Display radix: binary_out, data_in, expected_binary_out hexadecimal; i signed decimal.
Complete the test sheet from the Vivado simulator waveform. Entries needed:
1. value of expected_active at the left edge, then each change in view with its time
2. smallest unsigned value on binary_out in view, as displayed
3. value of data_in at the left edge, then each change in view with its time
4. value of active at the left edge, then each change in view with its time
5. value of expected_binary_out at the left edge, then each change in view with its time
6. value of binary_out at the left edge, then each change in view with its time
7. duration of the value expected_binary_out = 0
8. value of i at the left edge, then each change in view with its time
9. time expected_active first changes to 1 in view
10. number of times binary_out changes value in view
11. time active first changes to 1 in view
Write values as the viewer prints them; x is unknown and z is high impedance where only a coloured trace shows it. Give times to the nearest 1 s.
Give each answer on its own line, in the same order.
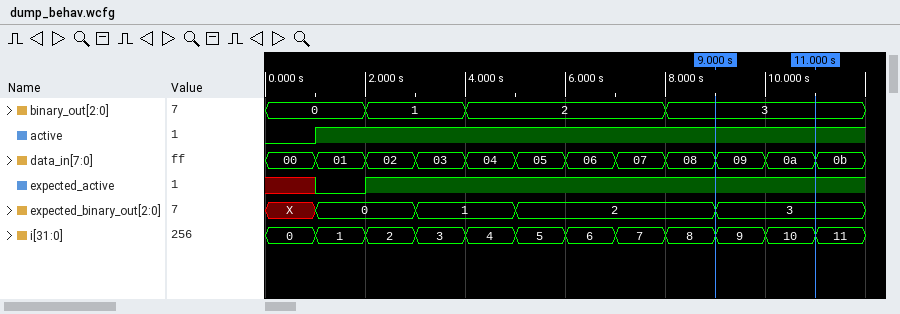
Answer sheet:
x, 0 at 1 s, 1 at 2 s
0
00, 01 at 1 s, 02 at 2 s, 03 at 3 s, 04 at 4 s, 05 at 5 s, 06 at 6 s, 07 at 7 s, 08 at 8 s, 09 at 9 s, 0a at 10 s, 0b at 11 s
0, 1 at 1 s
X, 0 at 1 s, 1 at 3 s, 2 at 5 s, 3 at 9 s
0, 1 at 2 s, 2 at 4 s, 3 at 8 s
2 s
0, 1 at 1 s, 2 at 2 s, 3 at 3 s, 4 at 4 s, 5 at 5 s, 6 at 6 s, 7 at 7 s, 8 at 8 s, 9 at 9 s, 10 at 10 s, 11 at 11 s
2 s
3
1 s
